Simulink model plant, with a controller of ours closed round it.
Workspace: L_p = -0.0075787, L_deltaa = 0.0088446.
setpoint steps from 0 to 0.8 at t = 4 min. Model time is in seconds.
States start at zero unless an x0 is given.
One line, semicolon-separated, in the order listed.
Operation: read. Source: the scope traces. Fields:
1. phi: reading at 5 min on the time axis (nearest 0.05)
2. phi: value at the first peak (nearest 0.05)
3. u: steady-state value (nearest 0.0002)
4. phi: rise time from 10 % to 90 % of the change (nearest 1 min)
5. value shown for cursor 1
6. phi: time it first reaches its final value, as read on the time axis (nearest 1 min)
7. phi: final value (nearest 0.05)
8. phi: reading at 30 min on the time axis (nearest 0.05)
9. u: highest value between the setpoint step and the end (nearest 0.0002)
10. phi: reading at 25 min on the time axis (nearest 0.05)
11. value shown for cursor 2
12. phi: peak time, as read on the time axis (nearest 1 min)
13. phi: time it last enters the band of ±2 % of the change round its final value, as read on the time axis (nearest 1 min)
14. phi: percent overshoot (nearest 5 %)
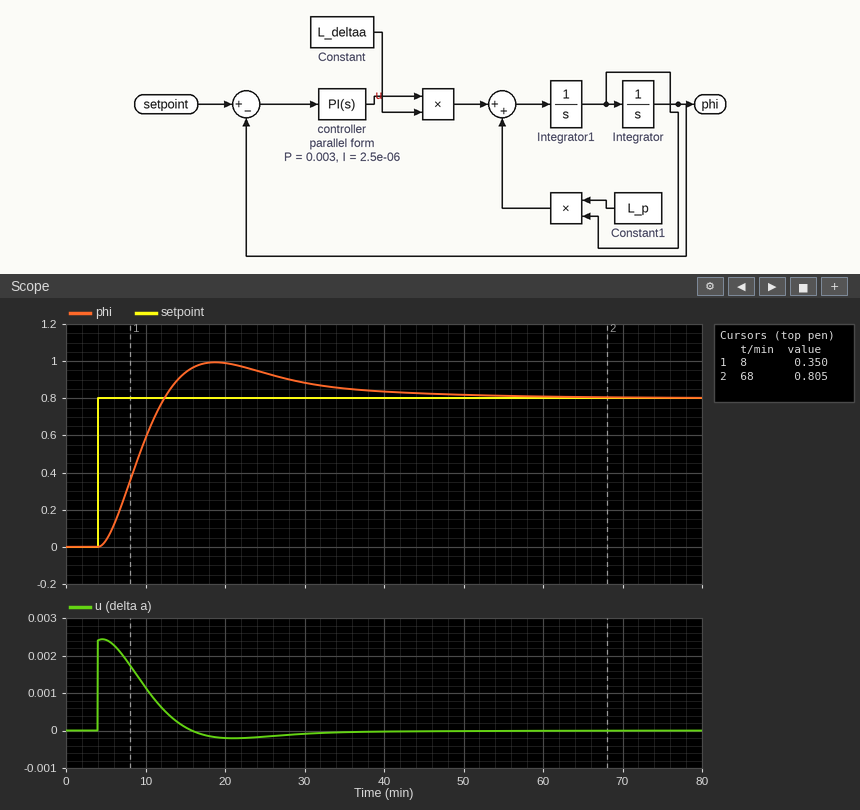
0.05; 1.00; 0.0000; 6 min; 0.350; 12 min; 0.80; 0.90; 0.0024; 0.95; 0.805; 19 min; 52 min; 25 %
